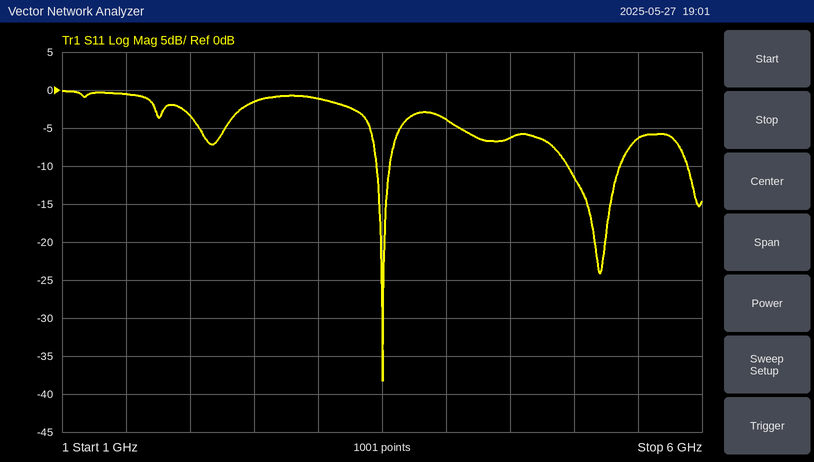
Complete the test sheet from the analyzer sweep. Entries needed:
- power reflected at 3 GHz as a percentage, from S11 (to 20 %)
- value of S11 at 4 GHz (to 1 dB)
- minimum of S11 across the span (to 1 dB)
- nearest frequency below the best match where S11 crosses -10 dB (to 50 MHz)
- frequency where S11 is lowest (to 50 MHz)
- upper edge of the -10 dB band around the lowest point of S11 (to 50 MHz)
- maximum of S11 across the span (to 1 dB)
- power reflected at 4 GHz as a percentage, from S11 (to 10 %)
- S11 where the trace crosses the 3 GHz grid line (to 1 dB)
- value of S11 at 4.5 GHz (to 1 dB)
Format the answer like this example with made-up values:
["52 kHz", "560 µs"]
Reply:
["80 %", "-4 dB", "-38 dB", "3.45 GHz", "3.50 GHz", "3.55 GHz", "0 dB", "40 %", "-1 dB", "-6 dB"]
